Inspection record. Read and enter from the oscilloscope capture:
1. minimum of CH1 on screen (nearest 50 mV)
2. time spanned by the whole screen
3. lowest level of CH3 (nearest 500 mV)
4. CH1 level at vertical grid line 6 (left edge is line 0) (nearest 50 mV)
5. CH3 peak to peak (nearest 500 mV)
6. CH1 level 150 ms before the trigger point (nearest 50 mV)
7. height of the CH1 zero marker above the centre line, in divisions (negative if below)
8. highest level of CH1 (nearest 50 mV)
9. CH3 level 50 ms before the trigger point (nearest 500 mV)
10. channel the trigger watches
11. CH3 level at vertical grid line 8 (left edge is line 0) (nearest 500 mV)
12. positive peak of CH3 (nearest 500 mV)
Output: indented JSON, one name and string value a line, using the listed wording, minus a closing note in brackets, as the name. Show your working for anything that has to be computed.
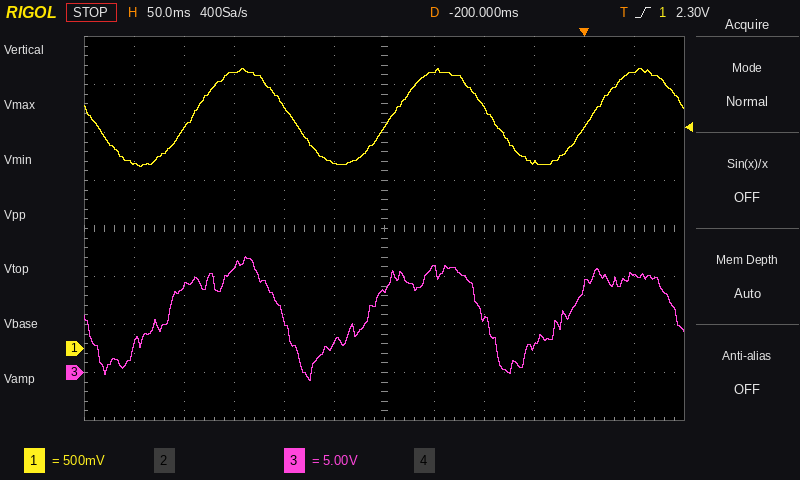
{
  "minimum of CH1 on screen": "1.90 V",
  "time spanned by the whole screen": "600 ms",
  "lowest level of CH3": "-1.0 V",
  "CH1 level at vertical grid line 6 (left edge is line 0)": "2.30 V",
  "CH3 peak to peak": "12.0 V − (-1.0 V) = 13.0 V",
  "CH1 level 150 ms before the trigger point": "2.90 V",
  "height of the CH1 zero marker above the centre line, in divisions": "-2.5 div",
  "highest level of CH1": "2.90 V",
  "CH3 level 50 ms before the trigger point": "2.5 V",
  "channel the trigger watches": "CH1",
  "CH3 level at vertical grid line 8 (left edge is line 0)": "5.5 V",
  "positive peak of CH3": "12.0 V"
}
